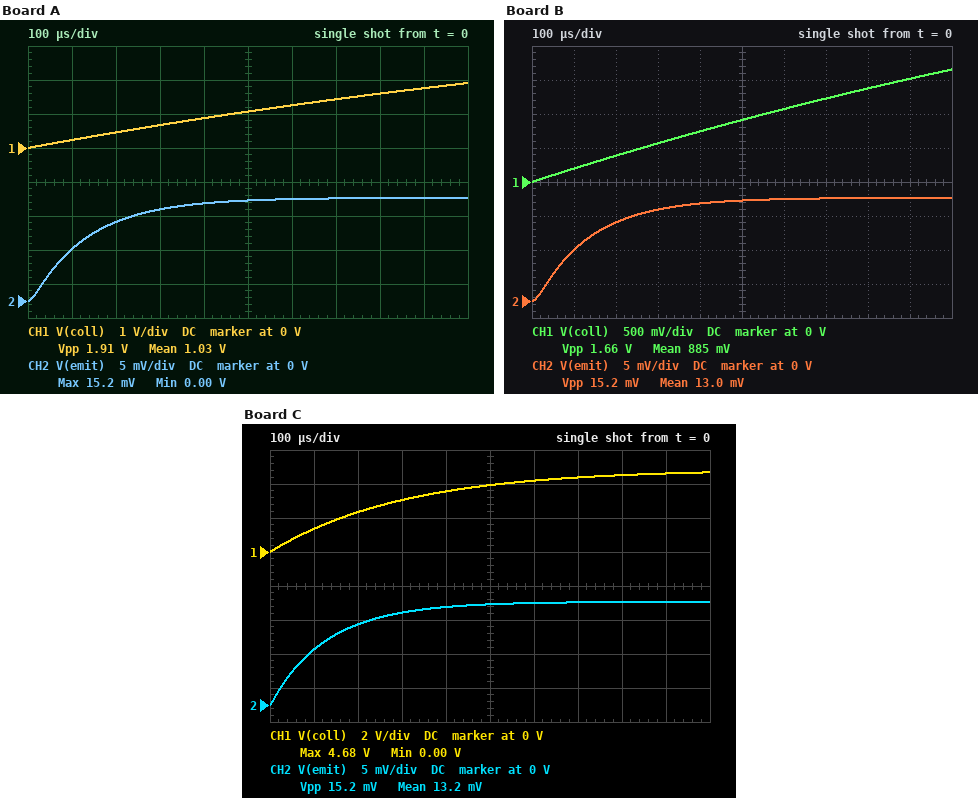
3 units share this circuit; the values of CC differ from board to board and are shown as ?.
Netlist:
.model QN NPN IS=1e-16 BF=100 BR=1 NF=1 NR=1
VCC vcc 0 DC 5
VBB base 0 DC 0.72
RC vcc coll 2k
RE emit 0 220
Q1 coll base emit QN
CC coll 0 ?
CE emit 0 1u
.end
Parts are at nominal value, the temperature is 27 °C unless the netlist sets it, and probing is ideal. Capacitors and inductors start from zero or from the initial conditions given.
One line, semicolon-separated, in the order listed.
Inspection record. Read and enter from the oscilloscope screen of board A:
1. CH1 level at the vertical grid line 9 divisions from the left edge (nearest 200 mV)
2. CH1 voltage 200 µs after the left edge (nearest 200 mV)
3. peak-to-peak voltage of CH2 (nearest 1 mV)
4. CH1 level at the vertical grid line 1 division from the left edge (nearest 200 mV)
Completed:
1.8 V; 400 mV; 15 mV; 200 mV
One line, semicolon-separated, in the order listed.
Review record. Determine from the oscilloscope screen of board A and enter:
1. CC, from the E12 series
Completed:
1 µF
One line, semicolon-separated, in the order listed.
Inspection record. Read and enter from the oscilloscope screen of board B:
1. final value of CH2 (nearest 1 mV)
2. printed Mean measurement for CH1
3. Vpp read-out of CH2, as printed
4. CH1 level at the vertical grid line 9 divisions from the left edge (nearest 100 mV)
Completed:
15 mV; 885 mV; 15.2 mV; 1.5 V
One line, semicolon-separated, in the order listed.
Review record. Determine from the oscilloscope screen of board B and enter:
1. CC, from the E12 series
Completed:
1.2 µF
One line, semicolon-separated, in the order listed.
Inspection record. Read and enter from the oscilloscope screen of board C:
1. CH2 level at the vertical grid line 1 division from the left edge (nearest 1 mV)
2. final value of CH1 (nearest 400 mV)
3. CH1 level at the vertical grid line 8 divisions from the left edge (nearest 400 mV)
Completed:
8 mV; 4.8 V; 4.4 V
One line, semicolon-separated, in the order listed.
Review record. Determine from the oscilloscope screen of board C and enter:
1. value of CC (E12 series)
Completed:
150 nF
